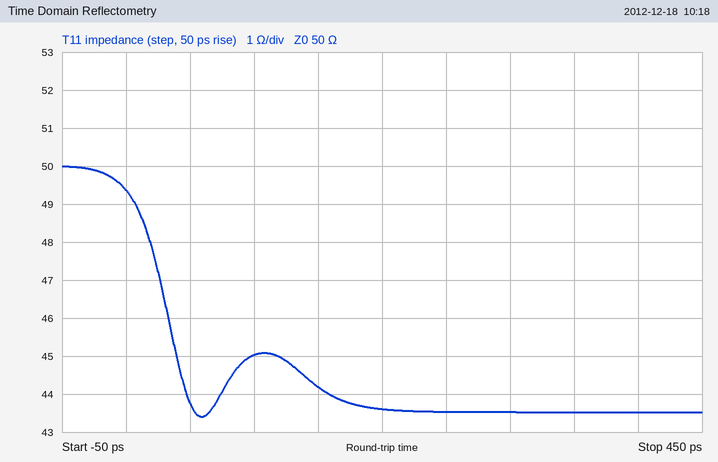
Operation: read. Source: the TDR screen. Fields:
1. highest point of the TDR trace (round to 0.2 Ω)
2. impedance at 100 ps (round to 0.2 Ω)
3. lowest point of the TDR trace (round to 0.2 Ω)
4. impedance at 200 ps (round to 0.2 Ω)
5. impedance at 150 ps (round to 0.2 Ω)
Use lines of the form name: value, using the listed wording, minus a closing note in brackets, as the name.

highest point of the TDR trace: 50.0 Ω
impedance at 100 ps: 45.0 Ω
lowest point of the TDR trace: 43.4 Ω
impedance at 200 ps: 43.6 Ω
impedance at 150 ps: 44.2 Ω
